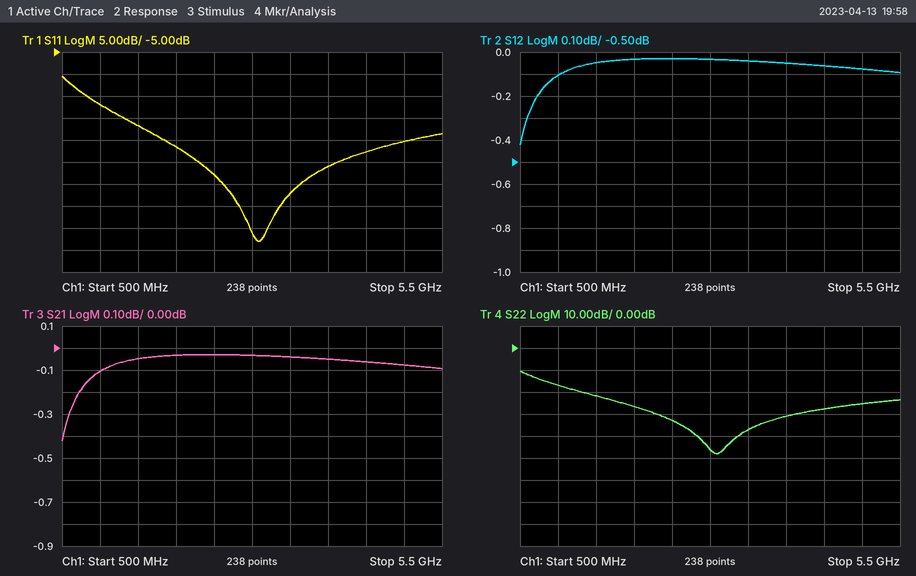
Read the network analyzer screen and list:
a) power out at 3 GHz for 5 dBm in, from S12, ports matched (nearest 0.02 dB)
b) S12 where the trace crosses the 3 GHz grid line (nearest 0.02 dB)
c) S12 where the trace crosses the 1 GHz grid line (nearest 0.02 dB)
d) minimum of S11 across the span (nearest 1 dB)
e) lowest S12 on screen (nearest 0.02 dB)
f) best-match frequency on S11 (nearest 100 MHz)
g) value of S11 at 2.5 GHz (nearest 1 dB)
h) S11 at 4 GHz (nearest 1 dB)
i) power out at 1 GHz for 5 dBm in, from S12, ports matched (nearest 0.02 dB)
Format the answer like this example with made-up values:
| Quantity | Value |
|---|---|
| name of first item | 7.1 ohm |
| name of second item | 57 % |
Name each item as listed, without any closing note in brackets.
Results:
| Quantity | Value |
|---|---|
| power out at 3 GHz for 5 dBm in, from S12, ports matched | 4.96 dBm |
| S12 where the trace crosses the 3 GHz grid line | -0.04 dB |
| S12 where the trace crosses the 1 GHz grid line | -0.10 dB |
| minimum of S11 across the span | -48 dB |
| lowest S12 on screen | -0.42 dB |
| best-match frequency on S11 | 3.1 GHz |
| value of S11 at 2.5 GHz | -33 dB |
| S11 at 4 GHz | -31 dB |
| power out at 1 GHz for 5 dBm in, from S12, ports matched | 4.90 dBm |
